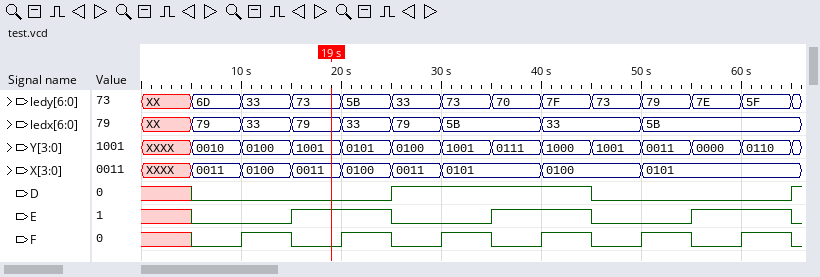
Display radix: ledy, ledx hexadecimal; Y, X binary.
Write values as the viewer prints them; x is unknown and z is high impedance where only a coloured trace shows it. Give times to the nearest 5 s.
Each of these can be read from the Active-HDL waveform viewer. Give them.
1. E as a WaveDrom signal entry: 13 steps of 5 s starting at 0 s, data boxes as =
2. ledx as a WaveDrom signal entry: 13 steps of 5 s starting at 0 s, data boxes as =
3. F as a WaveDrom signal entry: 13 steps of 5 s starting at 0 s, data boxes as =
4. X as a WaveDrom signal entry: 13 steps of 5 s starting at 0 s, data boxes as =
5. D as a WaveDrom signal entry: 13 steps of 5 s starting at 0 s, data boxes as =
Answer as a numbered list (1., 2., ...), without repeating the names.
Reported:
1. {name: 'E', wave: 'x0.1.0.1.0.1.'}
2. {name: 'ledx', wave: 'x======.=.=..', data: '79 33 79 33 79 5B 33 5B'}
3. {name: 'F', wave: 'x010101010101'}
4. {name: 'X', wave: 'x======.=.=..', data: '0011 0100 0011 0100 0011 0101 0100 0101'}
5. {name: 'D', wave: 'x0...1...0...'}
